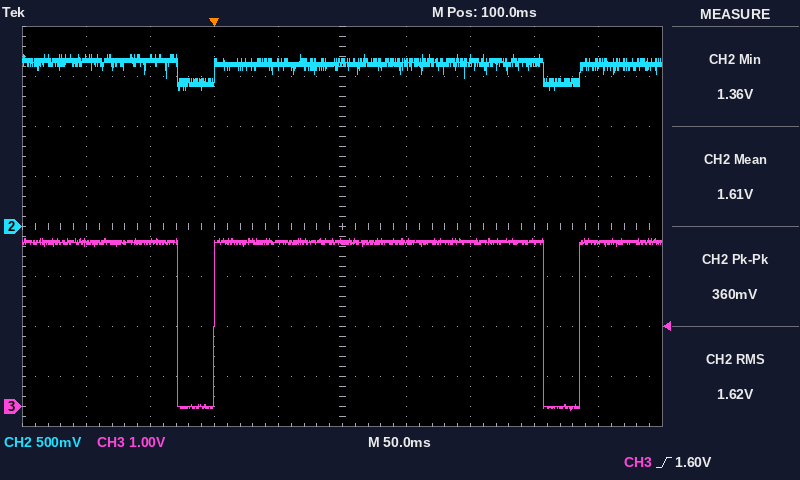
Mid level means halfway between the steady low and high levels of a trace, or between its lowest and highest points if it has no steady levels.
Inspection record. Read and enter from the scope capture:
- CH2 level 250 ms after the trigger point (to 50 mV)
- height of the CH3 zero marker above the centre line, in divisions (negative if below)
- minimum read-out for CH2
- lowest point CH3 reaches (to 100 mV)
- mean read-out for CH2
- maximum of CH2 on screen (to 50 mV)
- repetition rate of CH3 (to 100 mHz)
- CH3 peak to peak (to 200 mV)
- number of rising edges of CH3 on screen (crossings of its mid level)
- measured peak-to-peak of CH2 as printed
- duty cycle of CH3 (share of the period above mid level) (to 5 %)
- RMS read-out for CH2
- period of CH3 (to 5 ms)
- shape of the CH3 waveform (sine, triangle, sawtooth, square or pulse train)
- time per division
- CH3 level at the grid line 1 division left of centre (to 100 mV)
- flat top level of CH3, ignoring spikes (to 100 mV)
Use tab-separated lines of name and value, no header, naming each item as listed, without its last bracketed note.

CH2 level 250 ms after the trigger point	1.65 V
height of the CH3 zero marker above the centre line, in divisions	-3.6 div
minimum read-out for CH2	1.36 V
lowest point CH3 reaches	-100 mV
mean read-out for CH2	1.61 V
maximum of CH2 on screen	1.70 V
repetition rate of CH3	3.5 Hz
CH3 peak to peak	3.4 V
number of rising edges of CH3 on screen	2
measured peak-to-peak of CH2 as printed	360 mV
duty cycle of CH3 (share of the period above mid level)	90 %
RMS read-out for CH2	1.62 V
period of CH3	285 ms
shape of the CH3 waveform	pulse train
time per division	50 ms
CH3 level at the grid line 1 division left of centre	3.3 V
flat top level of CH3, ignoring spikes	3.3 V
